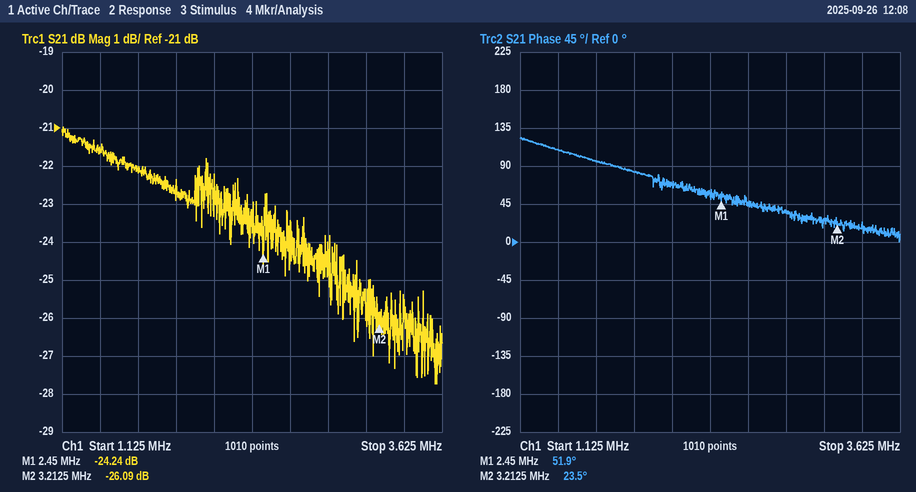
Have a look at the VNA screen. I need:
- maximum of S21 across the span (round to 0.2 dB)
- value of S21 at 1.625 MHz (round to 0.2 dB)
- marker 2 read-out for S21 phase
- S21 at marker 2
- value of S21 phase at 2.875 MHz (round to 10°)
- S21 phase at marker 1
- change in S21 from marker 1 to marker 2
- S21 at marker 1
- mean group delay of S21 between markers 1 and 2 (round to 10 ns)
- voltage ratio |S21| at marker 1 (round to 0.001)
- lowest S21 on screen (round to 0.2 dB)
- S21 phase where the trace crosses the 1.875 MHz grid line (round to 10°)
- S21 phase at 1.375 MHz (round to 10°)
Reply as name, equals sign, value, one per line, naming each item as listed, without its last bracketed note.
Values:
maximum of S21 across the span = -21.0 dB
value of S21 at 1.625 MHz = -22.0 dB
marker 2 read-out for S21 phase = 23.5°
S21 at marker 2 = -26.09 dB
value of S21 phase at 2.875 MHz = 40°
S21 phase at marker 1 = 51.9°
change in S21 from marker 1 to marker 2 = -1.85 dB
S21 at marker 1 = -24.24 dB
mean group delay of S21 between markers 1 and 2 = 100 ns
voltage ratio |S21| at marker 1 = 0.061
lowest S21 on screen = -27.8 dB
S21 phase where the trace crosses the 1.875 MHz grid line = 80°
S21 phase at 1.375 MHz = 110°
